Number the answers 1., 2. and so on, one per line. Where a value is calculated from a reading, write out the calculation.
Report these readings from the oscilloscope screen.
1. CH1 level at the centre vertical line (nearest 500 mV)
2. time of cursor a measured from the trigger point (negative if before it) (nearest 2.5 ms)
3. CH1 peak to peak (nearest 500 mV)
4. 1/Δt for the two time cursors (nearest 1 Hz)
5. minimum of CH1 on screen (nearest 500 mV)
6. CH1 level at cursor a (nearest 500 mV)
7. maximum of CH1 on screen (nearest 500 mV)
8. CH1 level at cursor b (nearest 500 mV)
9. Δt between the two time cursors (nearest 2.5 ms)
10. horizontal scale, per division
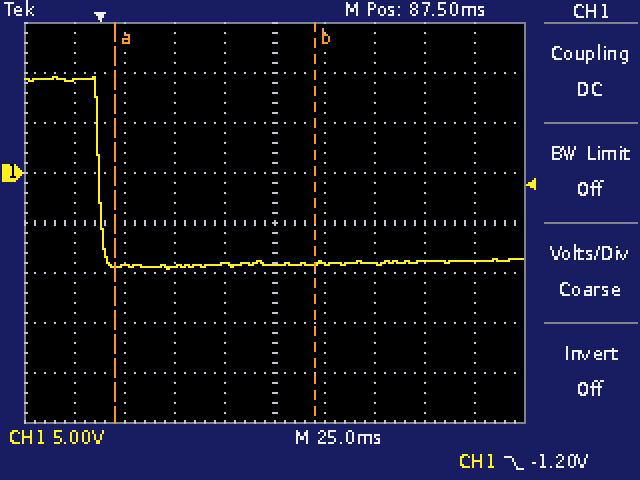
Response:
1. -9.0 V
2. +7.5 ms
3. 9.5 V − (-9.5 V) = 19.0 V
4. 1 / 100.0 ms ≈ 10 Hz
5. -9.5 V
6. -9.0 V
7. 9.5 V
8. -9.0 V
9. 100.0 ms
10. 25 ms
